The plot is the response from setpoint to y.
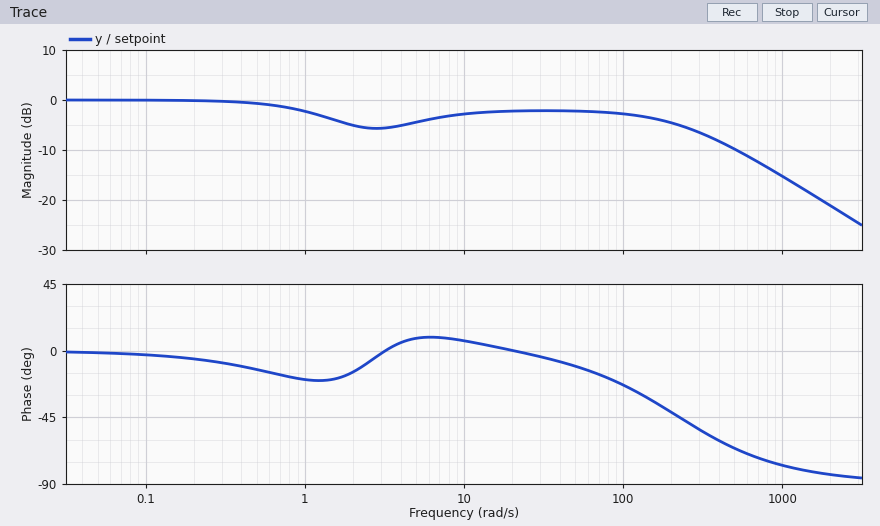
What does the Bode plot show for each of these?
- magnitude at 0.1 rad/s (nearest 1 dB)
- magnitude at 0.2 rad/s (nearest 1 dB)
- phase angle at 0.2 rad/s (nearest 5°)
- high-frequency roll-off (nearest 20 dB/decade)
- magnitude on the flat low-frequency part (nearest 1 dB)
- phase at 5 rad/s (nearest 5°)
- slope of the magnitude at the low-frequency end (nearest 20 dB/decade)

0 dB
0 dB
-5°
-20 dB/decade
0 dB
10°
0 dB/decade
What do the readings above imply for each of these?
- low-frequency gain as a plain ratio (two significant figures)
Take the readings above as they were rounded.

1.0
